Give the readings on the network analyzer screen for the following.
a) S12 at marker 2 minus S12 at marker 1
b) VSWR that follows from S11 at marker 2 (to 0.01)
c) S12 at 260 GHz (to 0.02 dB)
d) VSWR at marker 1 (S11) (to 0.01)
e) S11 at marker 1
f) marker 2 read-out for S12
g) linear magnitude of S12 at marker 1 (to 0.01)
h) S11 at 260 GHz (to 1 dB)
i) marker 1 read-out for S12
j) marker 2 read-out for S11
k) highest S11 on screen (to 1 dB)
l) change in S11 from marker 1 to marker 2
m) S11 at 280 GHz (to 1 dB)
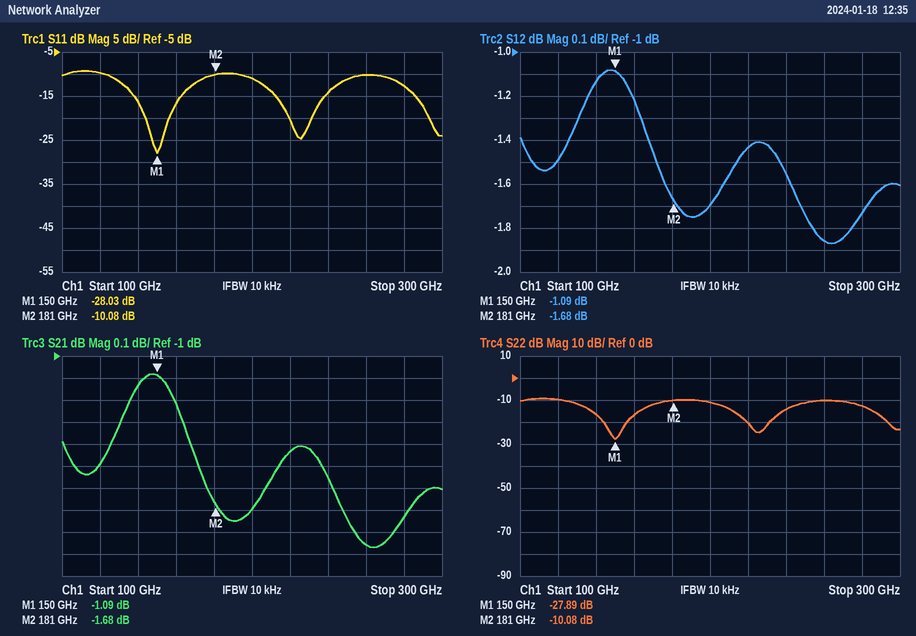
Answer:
-0.59 dB
1.91
-1.86 dB
1.08
-28.03 dB
-1.68 dB
0.88
-10 dB
-1.09 dB
-10.08 dB
-9 dB
17.95 dB
-13 dB
